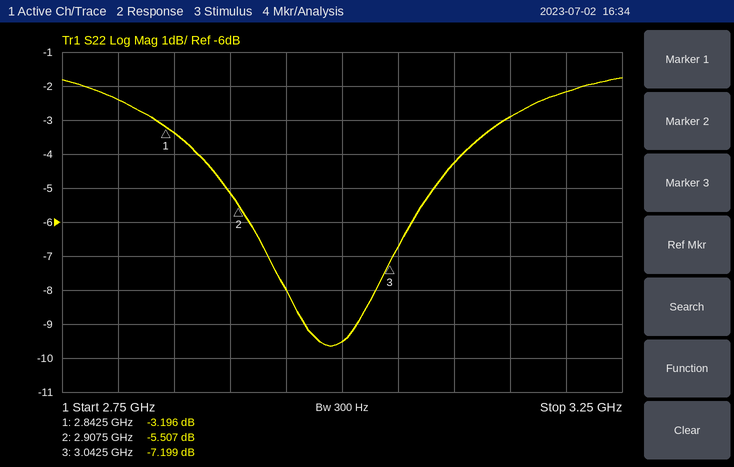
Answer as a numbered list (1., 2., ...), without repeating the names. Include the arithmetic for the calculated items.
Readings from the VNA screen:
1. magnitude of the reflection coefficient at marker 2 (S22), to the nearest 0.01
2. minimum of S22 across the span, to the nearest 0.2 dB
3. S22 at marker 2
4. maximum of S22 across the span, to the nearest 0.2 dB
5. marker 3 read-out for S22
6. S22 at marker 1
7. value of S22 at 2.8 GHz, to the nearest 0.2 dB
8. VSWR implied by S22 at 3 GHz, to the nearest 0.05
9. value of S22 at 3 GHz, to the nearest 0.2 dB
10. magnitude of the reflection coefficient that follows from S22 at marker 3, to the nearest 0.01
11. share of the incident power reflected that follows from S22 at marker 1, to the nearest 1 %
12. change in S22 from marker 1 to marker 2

1. 10^(-5.507/20) ≈ 0.53
2. -9.6 dB
3. -5.507 dB
4. -1.8 dB
5. -7.199 dB
6. -3.196 dB
7. -2.4 dB
8. |Γ| = 10^(-9.6/20) = 0.3311; VSWR = (1 + 0.3311)/(1 − 0.3311) ≈ 1.99, so 2.00 to the nearest 0.05
9. -9.6 dB
10. 10^(-7.199/20) ≈ 0.44
11. 10^(-3.196/10) ≈ 48 %
12. -5.507 − (-3.196) = -2.311 dB
